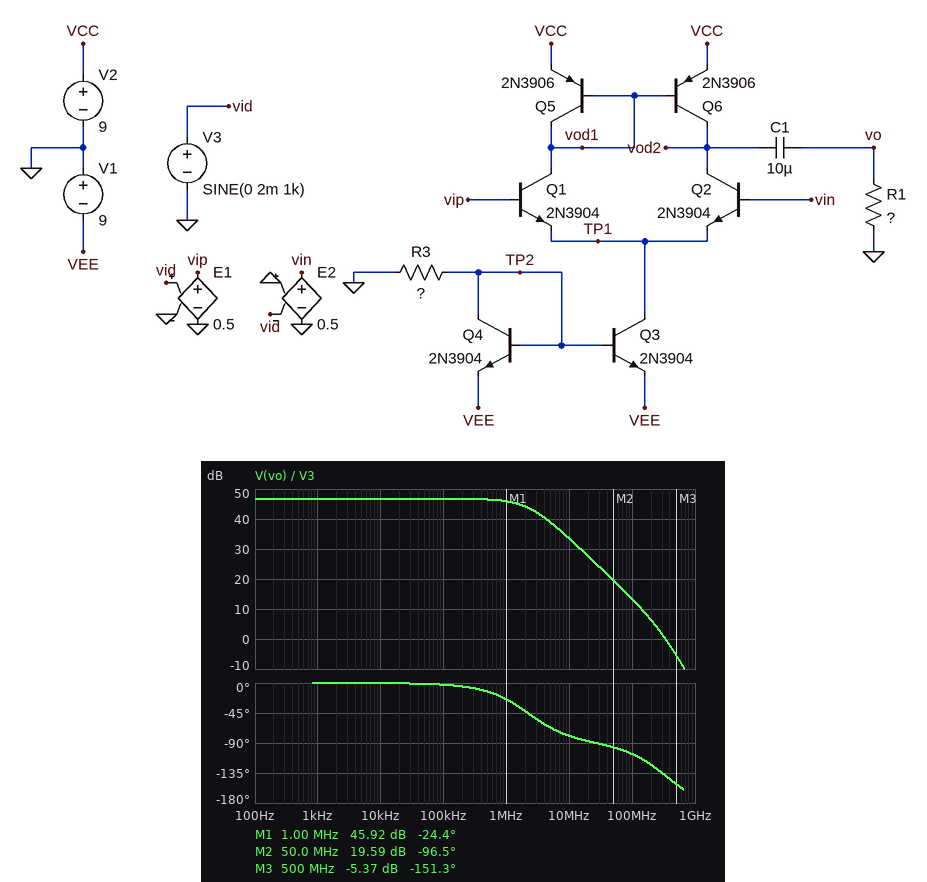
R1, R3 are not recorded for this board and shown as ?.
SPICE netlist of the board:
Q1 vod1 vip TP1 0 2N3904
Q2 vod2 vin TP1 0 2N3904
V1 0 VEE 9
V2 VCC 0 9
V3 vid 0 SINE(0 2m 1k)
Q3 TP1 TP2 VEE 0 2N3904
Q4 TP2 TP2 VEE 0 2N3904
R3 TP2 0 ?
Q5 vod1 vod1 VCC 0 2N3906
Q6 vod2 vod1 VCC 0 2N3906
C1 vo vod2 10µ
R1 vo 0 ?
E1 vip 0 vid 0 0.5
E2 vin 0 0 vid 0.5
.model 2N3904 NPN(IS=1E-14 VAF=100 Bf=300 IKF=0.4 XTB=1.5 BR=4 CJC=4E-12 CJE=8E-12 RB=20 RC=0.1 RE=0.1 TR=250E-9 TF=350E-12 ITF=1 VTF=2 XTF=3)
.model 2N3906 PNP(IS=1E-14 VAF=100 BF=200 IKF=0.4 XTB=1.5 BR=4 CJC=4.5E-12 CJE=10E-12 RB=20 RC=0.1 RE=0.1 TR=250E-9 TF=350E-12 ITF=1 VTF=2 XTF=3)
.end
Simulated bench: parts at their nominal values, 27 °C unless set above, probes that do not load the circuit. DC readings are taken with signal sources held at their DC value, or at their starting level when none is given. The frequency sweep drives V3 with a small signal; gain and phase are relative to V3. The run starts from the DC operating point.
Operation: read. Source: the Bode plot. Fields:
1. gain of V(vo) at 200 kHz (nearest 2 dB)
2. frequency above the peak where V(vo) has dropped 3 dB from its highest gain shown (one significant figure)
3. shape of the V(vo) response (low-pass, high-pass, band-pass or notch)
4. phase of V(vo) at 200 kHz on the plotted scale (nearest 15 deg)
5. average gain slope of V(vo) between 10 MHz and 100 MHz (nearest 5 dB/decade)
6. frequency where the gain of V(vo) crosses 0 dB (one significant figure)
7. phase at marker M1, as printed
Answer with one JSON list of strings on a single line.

["46 dB", "2 MHz", "low-pass", "0 deg", "-20 dB/decade", "300 MHz", "-24.4 deg"]
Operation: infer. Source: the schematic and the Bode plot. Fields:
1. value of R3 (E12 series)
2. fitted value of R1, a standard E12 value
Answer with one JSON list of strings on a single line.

["3.9 kΩ", "5.6 kΩ"]
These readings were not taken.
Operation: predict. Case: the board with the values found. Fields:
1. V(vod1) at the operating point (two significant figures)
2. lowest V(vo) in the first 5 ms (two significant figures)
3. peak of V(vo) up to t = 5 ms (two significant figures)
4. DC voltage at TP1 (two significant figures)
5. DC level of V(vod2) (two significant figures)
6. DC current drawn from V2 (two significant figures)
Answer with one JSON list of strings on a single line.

["8.3 V", "-430 mV", "430 mV", "-660 mV", "7.8 V", "2.3 mA"]
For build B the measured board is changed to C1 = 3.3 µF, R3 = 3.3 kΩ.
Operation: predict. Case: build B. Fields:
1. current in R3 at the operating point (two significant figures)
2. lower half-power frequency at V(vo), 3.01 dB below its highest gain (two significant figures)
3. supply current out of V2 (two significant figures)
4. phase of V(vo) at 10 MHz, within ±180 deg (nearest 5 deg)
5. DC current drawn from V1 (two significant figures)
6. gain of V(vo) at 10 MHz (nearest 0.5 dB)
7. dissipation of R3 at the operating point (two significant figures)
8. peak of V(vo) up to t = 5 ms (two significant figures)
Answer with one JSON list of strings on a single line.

["2.5 mA", "1.1 Hz", "2.7 mA", "-80 deg", "5.2 mA", "34.5 dB", "21 mW", "500 mV"]
